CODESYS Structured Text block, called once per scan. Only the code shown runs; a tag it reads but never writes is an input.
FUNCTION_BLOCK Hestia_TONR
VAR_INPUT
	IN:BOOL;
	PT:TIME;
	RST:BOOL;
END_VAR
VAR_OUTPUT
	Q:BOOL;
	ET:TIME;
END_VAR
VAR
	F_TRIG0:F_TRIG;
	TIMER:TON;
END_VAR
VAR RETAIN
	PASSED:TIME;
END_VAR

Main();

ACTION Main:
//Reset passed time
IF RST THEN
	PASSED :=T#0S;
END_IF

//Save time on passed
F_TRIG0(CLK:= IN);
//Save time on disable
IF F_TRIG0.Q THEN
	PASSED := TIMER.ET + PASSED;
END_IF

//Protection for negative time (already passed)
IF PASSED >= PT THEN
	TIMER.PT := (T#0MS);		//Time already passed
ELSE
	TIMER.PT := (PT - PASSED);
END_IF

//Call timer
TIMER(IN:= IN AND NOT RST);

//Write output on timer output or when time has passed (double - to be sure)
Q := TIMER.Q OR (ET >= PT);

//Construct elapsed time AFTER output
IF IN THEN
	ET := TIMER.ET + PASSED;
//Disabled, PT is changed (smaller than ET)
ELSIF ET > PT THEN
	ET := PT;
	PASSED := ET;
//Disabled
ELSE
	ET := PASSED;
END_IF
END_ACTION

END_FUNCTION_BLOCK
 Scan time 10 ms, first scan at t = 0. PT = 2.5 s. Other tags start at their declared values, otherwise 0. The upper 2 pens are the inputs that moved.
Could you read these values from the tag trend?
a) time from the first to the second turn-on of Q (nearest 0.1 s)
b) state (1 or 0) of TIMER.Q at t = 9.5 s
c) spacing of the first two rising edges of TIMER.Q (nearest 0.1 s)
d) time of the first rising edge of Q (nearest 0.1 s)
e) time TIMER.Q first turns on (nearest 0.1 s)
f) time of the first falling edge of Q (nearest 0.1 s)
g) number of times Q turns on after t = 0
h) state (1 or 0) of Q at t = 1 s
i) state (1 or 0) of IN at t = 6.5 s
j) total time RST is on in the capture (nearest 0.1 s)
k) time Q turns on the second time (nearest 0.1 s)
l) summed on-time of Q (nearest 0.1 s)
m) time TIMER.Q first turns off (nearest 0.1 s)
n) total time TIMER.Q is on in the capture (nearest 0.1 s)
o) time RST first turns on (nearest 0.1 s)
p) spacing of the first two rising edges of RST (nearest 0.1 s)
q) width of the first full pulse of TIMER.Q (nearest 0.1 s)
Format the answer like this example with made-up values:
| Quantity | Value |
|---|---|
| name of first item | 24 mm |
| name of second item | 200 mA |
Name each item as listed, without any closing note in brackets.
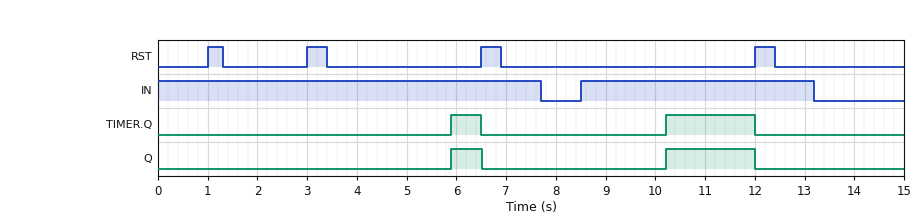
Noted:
| Quantity | Value |
|---|---|
| time from the first to the second turn-on of Q | 4.3 s |
| state (1 or 0) of TIMER.Q at t = 9.5 s | 0 |
| spacing of the first two rising edges of TIMER.Q | 4.3 s |
| time of the first rising edge of Q | 5.9 s |
| time TIMER.Q first turns on | 5.9 s |
| time of the first falling edge of Q | 6.5 s |
| number of times Q turns on after t = 0 | 2 |
| state (1 or 0) of Q at t = 1 s | 0 |
| state (1 or 0) of IN at t = 6.5 s | 1 |
| total time RST is on in the capture | 1.5 s |
| time Q turns on the second time | 10.2 s |
| summed on-time of Q | 2.4 s |
| time TIMER.Q first turns off | 6.5 s |
| total time TIMER.Q is on in the capture | 2.4 s |
| time RST first turns on | 1.0 s |
| spacing of the first two rising edges of RST | 2.0 s |
| width of the first full pulse of TIMER.Q | 0.6 s |
